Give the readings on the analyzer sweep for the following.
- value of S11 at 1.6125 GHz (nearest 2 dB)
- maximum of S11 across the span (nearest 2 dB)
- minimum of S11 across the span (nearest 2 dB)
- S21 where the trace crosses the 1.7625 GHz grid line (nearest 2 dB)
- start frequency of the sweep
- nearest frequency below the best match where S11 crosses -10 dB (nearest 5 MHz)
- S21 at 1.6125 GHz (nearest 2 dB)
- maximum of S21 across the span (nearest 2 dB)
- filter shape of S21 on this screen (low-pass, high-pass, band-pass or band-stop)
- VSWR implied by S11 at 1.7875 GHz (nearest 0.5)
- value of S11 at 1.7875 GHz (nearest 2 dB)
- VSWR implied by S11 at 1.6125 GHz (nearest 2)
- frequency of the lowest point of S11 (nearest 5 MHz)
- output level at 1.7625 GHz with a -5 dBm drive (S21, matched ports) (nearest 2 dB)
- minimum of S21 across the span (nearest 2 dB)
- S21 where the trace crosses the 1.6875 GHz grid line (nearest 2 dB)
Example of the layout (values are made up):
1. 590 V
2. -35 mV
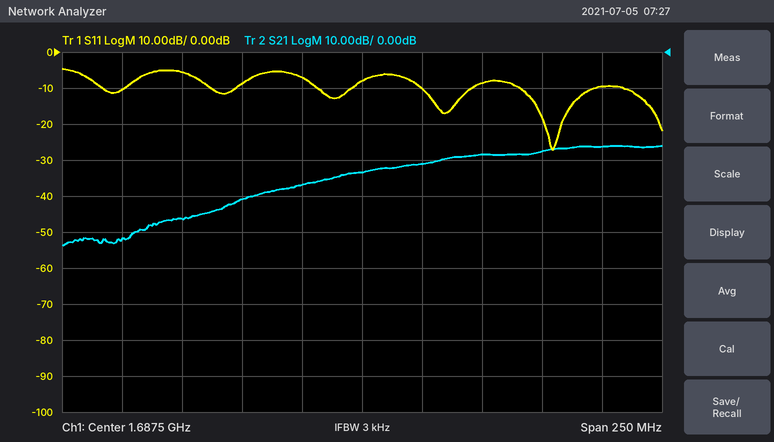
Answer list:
1. -6 dB
2. -4 dB
3. -28 dB
4. -28 dB
5. 1.5625 GHz
6. 1.755 GHz
7. -46 dB
8. -26 dB
9. high-pass
10. 2.0
11. -10 dB
12. 4
13. 1.765 GHz
14. -32 dBm
15. -54 dB
16. -34 dB
